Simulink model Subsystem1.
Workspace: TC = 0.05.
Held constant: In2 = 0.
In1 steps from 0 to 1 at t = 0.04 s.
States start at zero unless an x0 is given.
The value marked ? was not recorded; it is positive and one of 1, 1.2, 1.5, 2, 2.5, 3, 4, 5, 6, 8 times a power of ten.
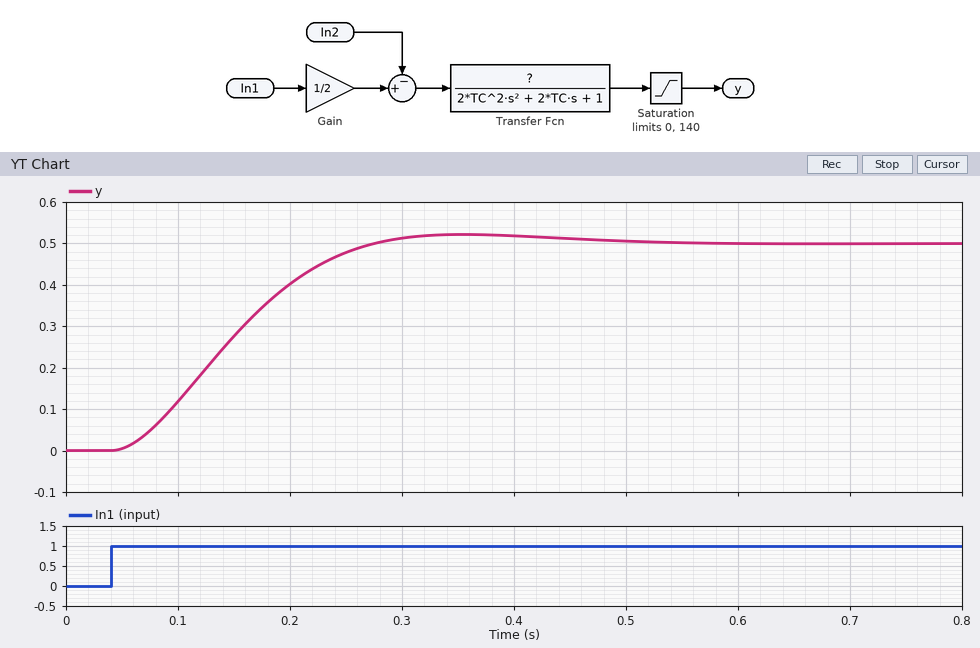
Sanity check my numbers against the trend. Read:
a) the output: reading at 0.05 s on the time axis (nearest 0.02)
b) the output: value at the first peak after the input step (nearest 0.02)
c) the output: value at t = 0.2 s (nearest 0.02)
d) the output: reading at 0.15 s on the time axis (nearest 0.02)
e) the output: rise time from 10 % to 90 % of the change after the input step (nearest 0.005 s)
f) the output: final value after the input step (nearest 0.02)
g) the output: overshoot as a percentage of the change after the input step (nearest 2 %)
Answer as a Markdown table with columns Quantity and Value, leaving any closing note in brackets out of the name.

| Quantity | Value |
|---|---|
| the output: reading at 0.05 s on the time axis | 0.00 |
| the output: value at the first peak after the input step | 0.52 |
| the output: value at t = 0.2 s | 0.40 |
| the output: reading at 0.15 s on the time axis | 0.28 |
| the output: rise time from 10 % to 90 % of the change after the input step | 0.150 s |
| the output: final value after the input step | 0.50 |
| the output: overshoot as a percentage of the change after the input step | 4 % |
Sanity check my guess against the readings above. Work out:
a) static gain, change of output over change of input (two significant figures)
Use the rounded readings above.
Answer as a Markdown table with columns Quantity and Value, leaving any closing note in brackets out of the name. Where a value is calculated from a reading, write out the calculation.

| Quantity | Value |
|---|---|
| static gain, change of output over change of input | (0.5 - 0) / (1 - 0) = 0.50 |
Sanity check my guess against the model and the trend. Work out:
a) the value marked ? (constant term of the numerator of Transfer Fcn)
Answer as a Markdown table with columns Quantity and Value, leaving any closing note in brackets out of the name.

| Quantity | Value |
|---|---|
| the value marked ? | 1 |
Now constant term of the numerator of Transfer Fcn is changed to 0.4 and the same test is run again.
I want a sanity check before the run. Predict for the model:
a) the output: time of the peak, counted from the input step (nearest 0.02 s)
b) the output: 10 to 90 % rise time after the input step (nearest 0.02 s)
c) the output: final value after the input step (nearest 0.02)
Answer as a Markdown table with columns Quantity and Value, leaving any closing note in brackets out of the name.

| Quantity | Value |
|---|---|
| the output: time of the peak, counted from the input step | 0.32 s |
| the output: 10 to 90 % rise time after the input step | 0.16 s |
| the output: final value after the input step | 0.20 |
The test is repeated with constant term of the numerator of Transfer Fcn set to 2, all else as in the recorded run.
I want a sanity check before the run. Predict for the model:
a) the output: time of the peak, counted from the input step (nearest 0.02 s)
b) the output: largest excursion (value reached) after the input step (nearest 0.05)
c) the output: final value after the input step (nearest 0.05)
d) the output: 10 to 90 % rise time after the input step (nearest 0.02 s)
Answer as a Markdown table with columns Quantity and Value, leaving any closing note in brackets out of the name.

| Quantity | Value |
|---|---|
| the output: time of the peak, counted from the input step | 0.32 s |
| the output: largest excursion (value reached) after the input step | 1.05 |
| the output: final value after the input step | 1.00 |
| the output: 10 to 90 % rise time after the input step | 0.16 s |
